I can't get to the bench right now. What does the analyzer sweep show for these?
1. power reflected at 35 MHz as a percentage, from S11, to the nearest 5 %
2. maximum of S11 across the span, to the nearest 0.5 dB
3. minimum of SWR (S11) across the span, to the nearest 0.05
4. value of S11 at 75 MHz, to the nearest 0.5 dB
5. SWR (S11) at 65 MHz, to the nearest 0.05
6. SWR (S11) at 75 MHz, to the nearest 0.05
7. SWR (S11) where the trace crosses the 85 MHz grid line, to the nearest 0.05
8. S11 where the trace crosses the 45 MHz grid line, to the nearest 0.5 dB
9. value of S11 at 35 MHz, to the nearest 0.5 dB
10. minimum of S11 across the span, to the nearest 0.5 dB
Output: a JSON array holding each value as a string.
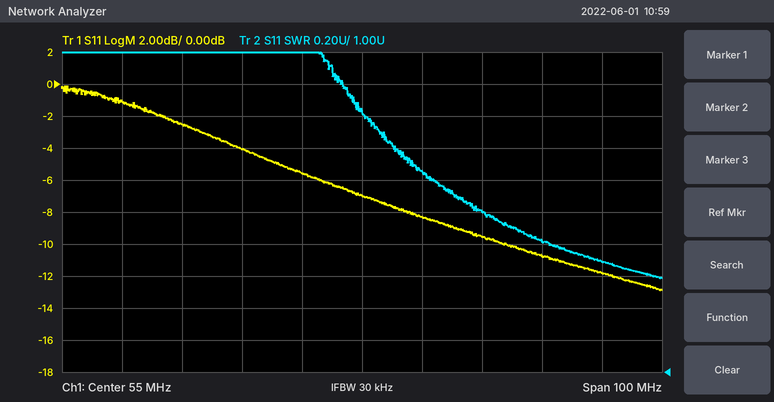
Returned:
["40 %", "0.0 dB", "1.60", "-9.5 dB", "2.25", "2.00", "1.80", "-5.5 dB", "-4.0 dB", "-13.0 dB"]
